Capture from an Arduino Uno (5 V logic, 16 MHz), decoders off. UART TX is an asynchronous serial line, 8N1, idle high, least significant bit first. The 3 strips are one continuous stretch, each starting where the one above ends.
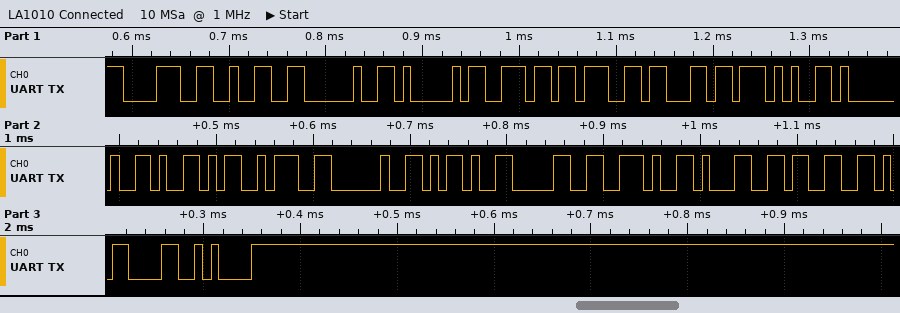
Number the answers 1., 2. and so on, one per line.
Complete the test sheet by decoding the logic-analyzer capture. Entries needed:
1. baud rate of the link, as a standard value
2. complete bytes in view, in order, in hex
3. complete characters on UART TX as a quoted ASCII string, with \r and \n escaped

1. 115200 baud
2. 38 32 20 41 6E 67 6C 65 20 59 3A 20 2D 30 2E 31 33 0D 0A
3. "82 Angle Y: -0.13\r\n"
